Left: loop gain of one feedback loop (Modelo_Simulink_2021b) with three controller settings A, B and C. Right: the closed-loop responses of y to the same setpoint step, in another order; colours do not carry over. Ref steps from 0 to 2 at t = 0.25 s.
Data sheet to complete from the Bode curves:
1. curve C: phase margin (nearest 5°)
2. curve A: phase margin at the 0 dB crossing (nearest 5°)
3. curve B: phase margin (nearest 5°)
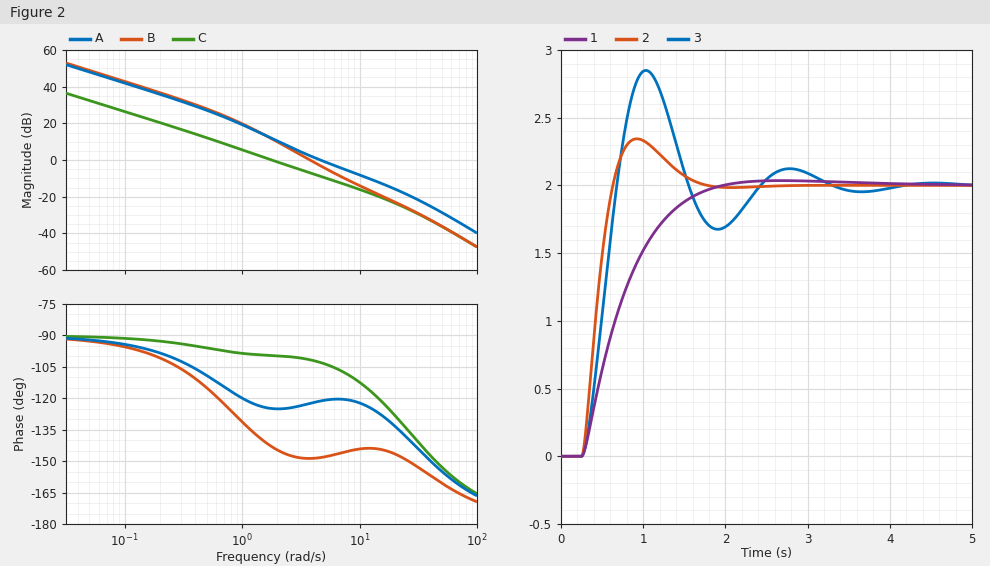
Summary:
80°
60°
30°
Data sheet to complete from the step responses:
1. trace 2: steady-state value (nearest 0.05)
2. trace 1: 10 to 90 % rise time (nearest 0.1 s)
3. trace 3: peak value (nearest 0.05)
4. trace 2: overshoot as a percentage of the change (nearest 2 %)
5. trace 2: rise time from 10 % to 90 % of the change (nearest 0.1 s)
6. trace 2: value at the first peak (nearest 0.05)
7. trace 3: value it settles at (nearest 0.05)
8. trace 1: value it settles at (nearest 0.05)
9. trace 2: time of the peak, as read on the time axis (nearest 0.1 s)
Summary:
2.00
1.0 s
2.85
18 %
0.3 s
2.35
2.00
2.00
0.9 s
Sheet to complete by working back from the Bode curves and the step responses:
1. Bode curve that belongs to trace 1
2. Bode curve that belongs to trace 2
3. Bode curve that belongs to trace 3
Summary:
C
A
B
